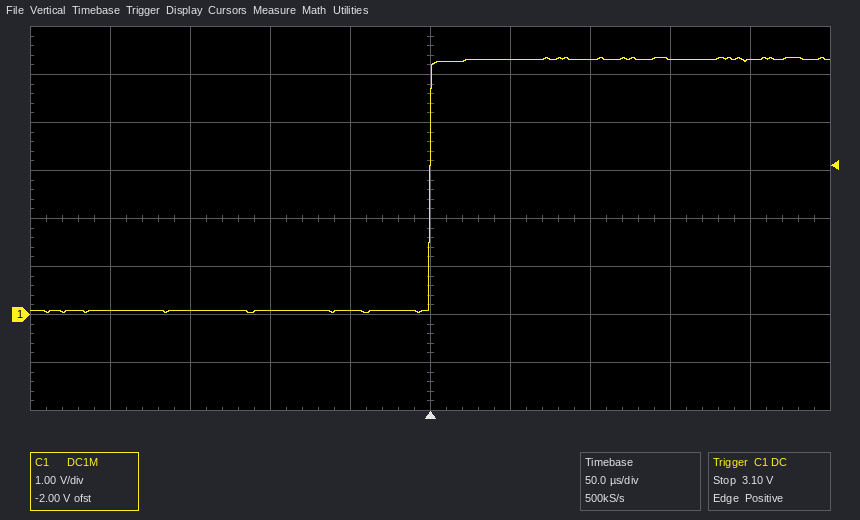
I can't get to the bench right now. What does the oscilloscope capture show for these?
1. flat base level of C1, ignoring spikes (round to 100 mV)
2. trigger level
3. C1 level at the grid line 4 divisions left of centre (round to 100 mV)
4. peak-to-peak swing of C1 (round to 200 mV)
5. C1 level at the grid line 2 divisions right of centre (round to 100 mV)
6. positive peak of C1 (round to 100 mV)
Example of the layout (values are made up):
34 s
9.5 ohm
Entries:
100 mV
3.10 V
100 mV
5.4 V
5.3 V
5.4 V
